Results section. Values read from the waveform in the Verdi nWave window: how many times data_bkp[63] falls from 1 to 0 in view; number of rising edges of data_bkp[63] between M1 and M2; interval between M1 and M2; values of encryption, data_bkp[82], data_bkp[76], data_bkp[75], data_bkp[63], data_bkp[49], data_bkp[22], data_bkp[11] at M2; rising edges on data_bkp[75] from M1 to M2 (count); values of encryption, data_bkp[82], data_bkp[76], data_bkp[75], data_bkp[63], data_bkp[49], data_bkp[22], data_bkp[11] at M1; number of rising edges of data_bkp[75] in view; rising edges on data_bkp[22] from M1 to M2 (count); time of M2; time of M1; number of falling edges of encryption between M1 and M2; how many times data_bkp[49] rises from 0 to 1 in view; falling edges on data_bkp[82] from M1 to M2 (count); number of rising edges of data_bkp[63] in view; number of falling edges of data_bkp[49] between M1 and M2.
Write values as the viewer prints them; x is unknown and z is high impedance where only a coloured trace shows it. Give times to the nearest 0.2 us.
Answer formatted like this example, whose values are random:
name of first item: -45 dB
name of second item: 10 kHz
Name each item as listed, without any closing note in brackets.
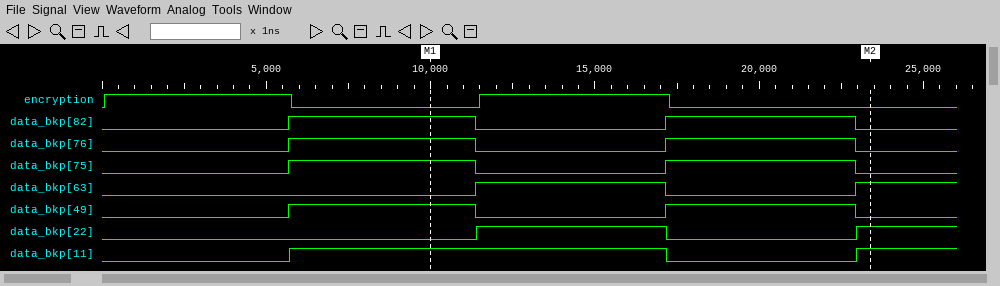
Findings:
how many times data_bkp[63] falls from 1 to 0 in view: 1
number of rising edges of data_bkp[63] between M1 and M2: 2
interval between M1 and M2: 13.4 us
values of encryption, data_bkp[82], data_bkp[76], data_bkp[75], data_bkp[63], data_bkp[49], data_bkp[22], data_bkp[11] at M2: encryption=0, data_bkp[82]=0, data_bkp[76]=0, data_bkp[75]=0, data_bkp[63]=1, data_bkp[49]=0, data_bkp[22]=1, data_bkp[11]=1
rising edges on data_bkp[75] from M1 to M2: 1
values of encryption, data_bkp[82], data_bkp[76], data_bkp[75], data_bkp[63], data_bkp[49], data_bkp[22], data_bkp[11] at M1: encryption=0, data_bkp[82]=1, data_bkp[76]=1, data_bkp[75]=1, data_bkp[63]=0, data_bkp[49]=1, data_bkp[22]=0, data_bkp[11]=1
number of rising edges of data_bkp[75] in view: 2
rising edges on data_bkp[22] from M1 to M2: 2
time of M2: 23.4 us
time of M1: 10 us
number of falling edges of encryption between M1 and M2: 1
how many times data_bkp[49] rises from 0 to 1 in view: 2
falling edges on data_bkp[82] from M1 to M2: 2
number of rising edges of data_bkp[63] in view: 2
number of falling edges of data_bkp[49] between M1 and M2: 2
